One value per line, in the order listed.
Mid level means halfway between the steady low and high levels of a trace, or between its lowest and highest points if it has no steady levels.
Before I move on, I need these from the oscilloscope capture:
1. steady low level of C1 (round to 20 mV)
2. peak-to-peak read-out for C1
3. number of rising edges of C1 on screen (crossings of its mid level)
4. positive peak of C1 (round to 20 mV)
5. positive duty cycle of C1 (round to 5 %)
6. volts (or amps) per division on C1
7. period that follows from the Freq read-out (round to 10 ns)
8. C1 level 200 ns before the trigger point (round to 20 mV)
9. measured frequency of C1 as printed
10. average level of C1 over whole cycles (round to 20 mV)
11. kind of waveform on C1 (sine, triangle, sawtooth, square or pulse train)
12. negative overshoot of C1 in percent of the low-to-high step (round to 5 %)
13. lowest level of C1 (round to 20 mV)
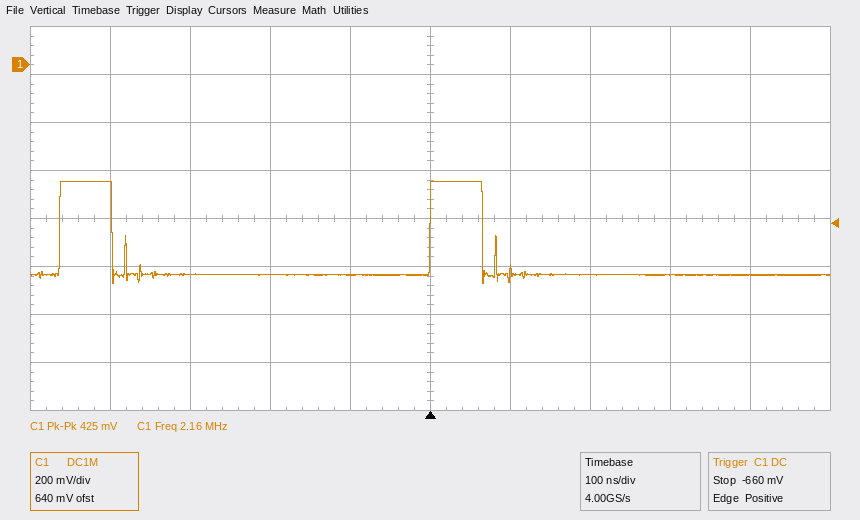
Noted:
-880 mV
425 mV
2
-480 mV
15 %
200 mV
460 ns
-880 mV
2.16 MHz
-820 mV
pulse train
10 %
-920 mV
